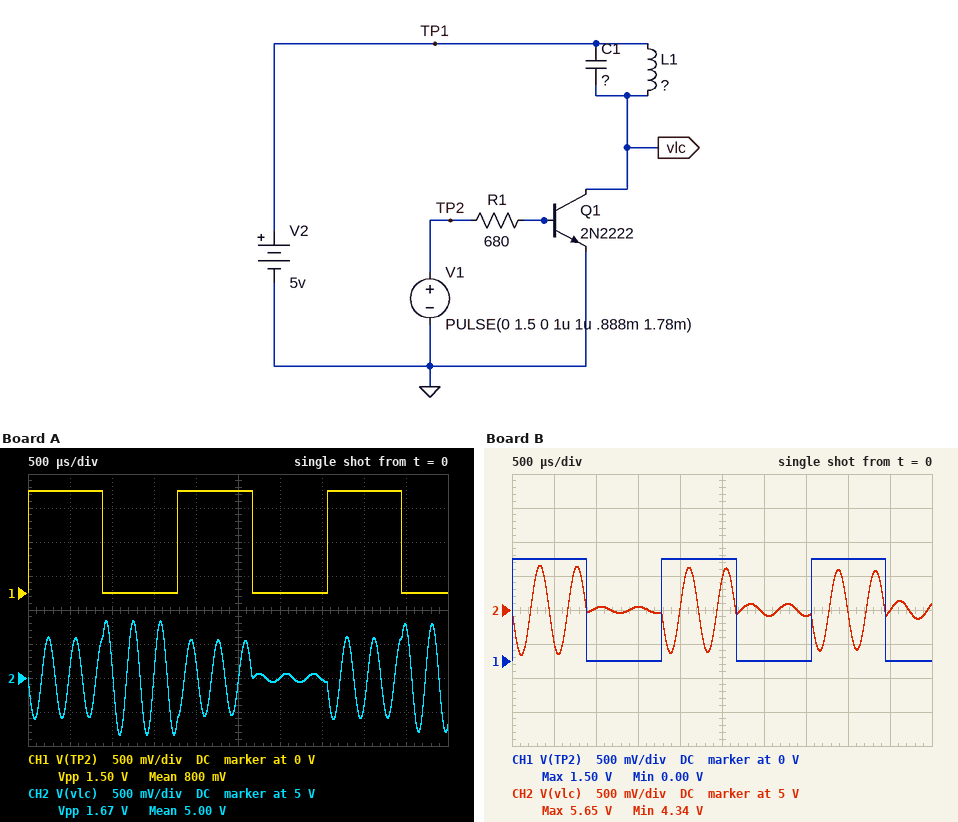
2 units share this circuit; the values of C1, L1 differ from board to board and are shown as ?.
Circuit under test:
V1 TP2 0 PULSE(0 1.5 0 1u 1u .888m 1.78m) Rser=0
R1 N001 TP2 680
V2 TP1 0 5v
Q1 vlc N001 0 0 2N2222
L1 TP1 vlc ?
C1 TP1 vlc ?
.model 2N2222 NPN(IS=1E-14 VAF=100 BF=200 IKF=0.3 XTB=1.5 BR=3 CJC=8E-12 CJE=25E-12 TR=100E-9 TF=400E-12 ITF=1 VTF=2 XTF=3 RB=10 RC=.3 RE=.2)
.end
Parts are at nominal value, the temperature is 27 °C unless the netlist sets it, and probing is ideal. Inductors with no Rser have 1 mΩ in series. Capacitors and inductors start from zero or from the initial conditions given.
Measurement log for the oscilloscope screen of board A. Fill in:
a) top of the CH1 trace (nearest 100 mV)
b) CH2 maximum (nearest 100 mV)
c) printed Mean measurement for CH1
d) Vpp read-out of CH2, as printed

1.5 V
5.8 V
800 mV
1.67 V
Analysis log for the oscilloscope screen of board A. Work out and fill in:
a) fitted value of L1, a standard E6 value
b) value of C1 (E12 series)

220 µH
12 µF
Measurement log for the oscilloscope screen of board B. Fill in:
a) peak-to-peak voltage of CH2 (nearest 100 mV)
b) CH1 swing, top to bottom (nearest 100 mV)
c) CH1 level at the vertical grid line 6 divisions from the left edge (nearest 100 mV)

1.3 V
1.5 V
0 V
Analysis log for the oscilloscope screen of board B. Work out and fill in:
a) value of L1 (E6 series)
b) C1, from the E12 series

330 µH
15 µF
